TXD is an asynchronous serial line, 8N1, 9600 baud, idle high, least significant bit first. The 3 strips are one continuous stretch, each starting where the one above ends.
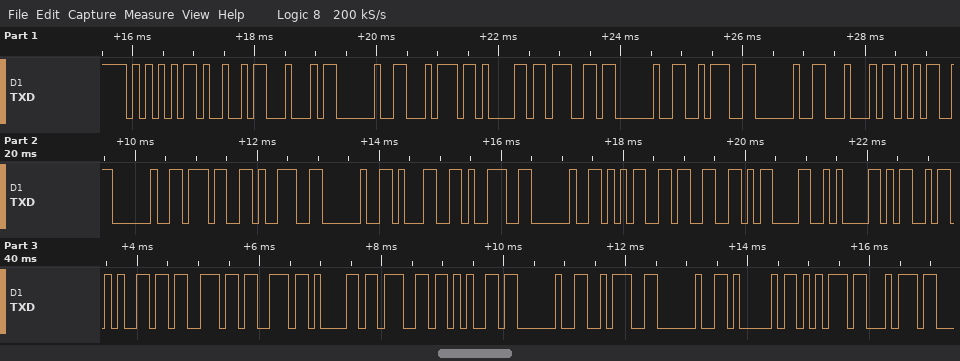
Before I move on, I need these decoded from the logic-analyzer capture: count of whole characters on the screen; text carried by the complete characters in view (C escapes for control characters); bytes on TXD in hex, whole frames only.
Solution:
36
"UID tag : D5 79 19 53\r\nMessage : Aut"
55 49 44 20 74 61 67 20 3A 20 44 35 20 37 39 20 31 39 20 35 33 0D 0A 4D 65 73 73 61 67 65 20 3A 20 41 75 74
